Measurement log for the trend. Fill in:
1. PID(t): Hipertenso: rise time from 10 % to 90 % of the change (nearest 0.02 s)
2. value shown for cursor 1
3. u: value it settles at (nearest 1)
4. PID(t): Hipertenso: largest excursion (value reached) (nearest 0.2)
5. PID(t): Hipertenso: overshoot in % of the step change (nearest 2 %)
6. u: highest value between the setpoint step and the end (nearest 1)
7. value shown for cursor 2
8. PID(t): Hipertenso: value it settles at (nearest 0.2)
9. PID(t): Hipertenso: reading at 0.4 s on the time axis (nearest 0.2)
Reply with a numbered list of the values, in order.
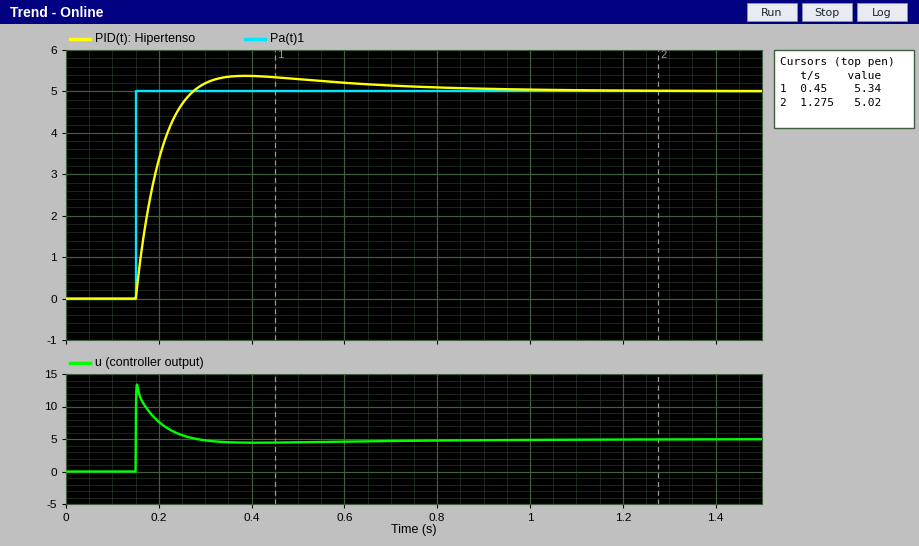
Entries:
1. 0.08 s
2. 5.34
3. 5
4. 5.4
5. 8 %
6. 13
7. 5.02
8. 5.0
9. 5.4
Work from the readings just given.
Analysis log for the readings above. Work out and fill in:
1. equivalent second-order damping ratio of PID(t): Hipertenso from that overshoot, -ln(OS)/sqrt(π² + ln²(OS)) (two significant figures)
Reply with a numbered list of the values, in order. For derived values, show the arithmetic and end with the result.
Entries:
1. ln(0.08) = -2.526; 2.526 / sqrt(9.870 + 6.379) = 0.63
